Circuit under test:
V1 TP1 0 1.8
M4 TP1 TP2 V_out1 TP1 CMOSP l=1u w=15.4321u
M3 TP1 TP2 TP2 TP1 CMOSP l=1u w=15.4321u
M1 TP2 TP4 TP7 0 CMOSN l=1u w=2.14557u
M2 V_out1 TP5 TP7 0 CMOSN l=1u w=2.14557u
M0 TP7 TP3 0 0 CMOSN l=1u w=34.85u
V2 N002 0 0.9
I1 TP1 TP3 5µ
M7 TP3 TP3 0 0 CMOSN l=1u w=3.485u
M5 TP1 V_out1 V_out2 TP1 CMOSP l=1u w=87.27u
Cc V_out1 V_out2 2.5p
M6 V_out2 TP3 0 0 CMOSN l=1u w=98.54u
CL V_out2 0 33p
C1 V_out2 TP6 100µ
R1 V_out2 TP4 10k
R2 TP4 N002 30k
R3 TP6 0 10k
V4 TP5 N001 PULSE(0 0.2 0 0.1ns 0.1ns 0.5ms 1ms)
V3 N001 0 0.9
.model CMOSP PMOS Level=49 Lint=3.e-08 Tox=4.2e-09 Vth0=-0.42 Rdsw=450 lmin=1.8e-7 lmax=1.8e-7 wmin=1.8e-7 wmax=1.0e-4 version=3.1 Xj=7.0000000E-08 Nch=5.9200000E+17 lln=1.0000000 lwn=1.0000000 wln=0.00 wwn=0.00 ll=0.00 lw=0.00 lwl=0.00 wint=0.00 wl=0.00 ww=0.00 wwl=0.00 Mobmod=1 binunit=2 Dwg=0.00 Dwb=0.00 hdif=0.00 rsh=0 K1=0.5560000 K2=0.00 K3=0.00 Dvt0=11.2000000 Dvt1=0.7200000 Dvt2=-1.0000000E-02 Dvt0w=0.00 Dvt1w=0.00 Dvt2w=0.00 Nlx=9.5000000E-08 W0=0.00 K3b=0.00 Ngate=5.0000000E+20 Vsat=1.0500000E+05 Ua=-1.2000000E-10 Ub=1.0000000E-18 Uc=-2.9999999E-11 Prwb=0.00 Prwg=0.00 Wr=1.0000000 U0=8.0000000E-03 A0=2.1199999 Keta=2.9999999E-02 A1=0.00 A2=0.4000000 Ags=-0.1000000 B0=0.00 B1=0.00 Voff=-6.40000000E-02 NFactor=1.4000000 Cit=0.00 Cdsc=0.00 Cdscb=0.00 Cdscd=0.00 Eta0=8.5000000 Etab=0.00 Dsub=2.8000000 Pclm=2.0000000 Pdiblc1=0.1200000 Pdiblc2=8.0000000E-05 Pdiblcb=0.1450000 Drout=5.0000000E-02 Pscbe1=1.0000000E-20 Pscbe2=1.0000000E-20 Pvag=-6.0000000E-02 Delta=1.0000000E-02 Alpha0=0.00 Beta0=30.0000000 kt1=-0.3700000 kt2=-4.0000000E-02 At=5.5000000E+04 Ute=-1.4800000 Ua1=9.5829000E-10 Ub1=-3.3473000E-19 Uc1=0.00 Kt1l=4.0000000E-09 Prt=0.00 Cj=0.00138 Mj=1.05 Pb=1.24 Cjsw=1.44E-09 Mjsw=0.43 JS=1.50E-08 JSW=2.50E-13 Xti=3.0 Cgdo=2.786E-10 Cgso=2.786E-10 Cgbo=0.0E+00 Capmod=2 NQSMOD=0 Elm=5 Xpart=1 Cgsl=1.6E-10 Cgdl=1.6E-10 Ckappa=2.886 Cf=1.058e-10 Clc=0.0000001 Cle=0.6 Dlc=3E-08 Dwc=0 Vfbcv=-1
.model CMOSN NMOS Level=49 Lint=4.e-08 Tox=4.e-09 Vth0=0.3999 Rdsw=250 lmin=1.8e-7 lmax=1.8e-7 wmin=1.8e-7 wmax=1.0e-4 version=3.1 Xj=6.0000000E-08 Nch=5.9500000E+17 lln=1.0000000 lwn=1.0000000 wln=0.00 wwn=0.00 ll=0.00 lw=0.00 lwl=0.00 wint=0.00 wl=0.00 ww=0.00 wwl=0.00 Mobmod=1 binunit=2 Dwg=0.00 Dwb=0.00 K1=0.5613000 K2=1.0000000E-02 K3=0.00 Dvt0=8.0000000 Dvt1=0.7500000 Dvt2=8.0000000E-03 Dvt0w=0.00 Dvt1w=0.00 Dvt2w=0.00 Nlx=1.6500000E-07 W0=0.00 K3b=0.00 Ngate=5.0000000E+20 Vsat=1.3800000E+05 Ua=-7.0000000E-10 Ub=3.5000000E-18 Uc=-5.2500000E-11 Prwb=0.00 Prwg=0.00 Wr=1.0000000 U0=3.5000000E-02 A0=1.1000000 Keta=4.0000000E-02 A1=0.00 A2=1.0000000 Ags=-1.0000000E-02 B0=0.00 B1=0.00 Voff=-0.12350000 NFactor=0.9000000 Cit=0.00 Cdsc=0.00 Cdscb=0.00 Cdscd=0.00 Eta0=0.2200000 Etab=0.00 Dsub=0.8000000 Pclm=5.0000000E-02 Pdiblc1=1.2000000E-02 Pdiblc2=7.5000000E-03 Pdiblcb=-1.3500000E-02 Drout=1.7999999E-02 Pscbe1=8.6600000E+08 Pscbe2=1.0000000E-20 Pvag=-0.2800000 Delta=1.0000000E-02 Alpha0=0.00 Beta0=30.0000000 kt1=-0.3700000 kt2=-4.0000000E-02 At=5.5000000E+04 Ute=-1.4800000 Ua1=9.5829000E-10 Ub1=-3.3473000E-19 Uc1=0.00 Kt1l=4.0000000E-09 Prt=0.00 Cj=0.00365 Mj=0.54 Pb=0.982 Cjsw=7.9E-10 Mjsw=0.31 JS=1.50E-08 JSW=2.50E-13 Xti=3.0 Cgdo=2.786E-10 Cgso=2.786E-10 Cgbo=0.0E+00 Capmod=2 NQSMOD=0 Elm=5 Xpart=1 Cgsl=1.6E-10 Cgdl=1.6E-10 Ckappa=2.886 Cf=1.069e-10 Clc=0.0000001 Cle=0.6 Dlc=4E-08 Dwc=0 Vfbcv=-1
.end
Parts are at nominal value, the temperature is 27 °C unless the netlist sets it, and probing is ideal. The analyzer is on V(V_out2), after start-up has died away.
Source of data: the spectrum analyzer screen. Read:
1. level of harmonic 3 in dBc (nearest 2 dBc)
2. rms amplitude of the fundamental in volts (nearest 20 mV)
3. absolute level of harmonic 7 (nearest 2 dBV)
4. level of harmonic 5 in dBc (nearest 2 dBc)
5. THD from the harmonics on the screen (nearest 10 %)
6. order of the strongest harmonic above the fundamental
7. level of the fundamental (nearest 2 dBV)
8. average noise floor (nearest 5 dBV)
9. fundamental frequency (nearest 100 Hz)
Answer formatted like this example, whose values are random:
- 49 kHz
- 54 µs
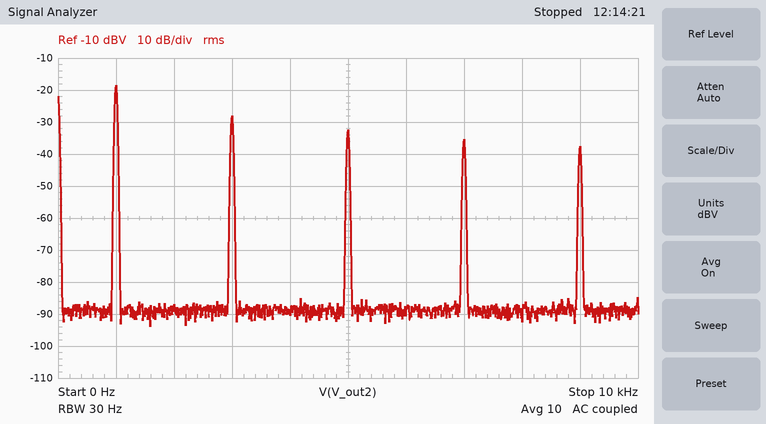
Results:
- -10 dBc
- 120 mV
- -36 dBV
- -14 dBc
- 40 %
- 3
- -18 dBV
- -90 dBV
- 1.0 kHz
